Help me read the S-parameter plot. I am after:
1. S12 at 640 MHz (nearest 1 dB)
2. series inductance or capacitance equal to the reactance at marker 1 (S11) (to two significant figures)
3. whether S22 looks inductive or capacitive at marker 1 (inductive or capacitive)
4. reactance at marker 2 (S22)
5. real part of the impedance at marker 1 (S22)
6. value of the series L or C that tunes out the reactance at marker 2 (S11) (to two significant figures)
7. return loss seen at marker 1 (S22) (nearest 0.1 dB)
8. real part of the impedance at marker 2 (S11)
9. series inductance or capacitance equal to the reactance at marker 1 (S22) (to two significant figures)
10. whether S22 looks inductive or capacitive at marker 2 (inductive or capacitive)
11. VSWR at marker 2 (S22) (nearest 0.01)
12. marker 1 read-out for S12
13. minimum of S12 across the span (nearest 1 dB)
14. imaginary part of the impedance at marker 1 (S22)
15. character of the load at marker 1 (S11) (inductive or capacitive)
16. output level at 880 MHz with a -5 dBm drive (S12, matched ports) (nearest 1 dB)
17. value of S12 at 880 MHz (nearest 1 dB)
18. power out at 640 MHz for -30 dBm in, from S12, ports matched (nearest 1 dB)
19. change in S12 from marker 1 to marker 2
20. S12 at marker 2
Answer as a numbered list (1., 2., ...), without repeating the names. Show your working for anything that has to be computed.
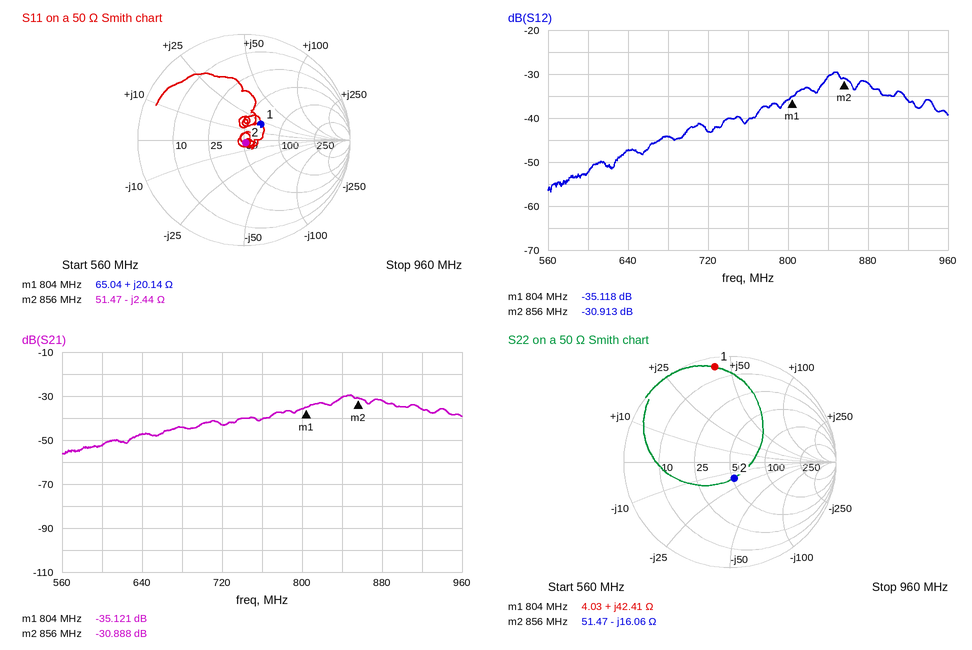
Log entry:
1. -47 dB
2. L = 20.14 Ω/(2π × 804 MHz) ≈ 4.0 nH
3. inductive
4. -16.06 Ω
5. 4.03 Ω
6. L = 2.44 Ω/(2π × 856 MHz) ≈ 454 pH, so 450 pH to two significant figures
7. 0.8 dB
8. 51.47 Ω
9. L = 42.41 Ω/(2π × 804 MHz) ≈ 8.4 nH
10. capacitive
11. 1.37
12. -35.118 dB
13. -57 dB
14. +42.41 Ω
15. inductive
16. -5 dBm + (-32 dB) = -37 dBm
17. -32 dB
18. -30 dBm + (-47 dB) = -77 dBm
19. -30.913 − (-35.118) = 4.205 dB
20. -30.913 dB
